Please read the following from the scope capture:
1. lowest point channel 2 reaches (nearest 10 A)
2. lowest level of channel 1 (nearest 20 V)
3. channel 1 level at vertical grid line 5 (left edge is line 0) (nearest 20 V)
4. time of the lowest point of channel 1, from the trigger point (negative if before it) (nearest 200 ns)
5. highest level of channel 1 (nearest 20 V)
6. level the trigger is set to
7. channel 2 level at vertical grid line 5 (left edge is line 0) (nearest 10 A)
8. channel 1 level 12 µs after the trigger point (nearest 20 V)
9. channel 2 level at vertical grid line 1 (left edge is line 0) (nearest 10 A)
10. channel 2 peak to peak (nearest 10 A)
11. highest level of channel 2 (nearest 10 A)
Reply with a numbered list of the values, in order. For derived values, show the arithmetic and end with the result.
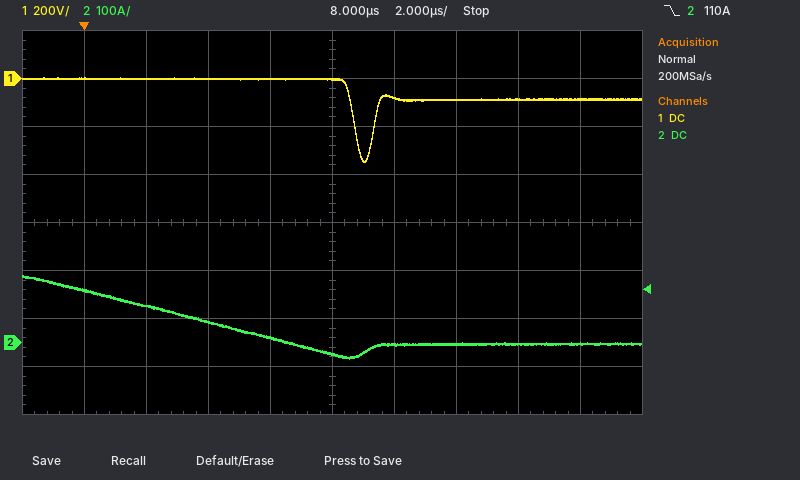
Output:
1. -30 A
2. -340 V
3. 0 V
4. +9.0 µs
5. 0 V
6. 110 A
7. -20 A
8. -80 V
9. 110 A
10. 140 A − (-30 A) = 170 A
11. 140 A
